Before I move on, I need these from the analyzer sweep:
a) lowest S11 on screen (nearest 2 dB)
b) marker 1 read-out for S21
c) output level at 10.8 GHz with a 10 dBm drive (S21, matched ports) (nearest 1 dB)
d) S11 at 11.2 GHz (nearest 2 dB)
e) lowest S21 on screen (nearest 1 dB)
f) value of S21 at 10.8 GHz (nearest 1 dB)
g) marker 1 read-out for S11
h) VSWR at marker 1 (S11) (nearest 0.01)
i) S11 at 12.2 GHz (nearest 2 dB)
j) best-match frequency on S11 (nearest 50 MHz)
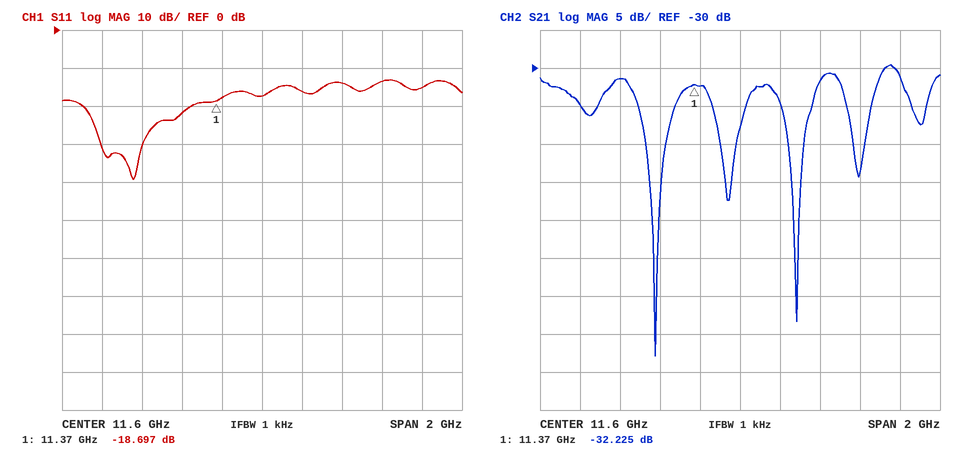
-40 dB
-32.225 dB
-25 dBm
-22 dB
-68 dB
-35 dB
-18.697 dB
1.26
-14 dB
10.95 GHz
